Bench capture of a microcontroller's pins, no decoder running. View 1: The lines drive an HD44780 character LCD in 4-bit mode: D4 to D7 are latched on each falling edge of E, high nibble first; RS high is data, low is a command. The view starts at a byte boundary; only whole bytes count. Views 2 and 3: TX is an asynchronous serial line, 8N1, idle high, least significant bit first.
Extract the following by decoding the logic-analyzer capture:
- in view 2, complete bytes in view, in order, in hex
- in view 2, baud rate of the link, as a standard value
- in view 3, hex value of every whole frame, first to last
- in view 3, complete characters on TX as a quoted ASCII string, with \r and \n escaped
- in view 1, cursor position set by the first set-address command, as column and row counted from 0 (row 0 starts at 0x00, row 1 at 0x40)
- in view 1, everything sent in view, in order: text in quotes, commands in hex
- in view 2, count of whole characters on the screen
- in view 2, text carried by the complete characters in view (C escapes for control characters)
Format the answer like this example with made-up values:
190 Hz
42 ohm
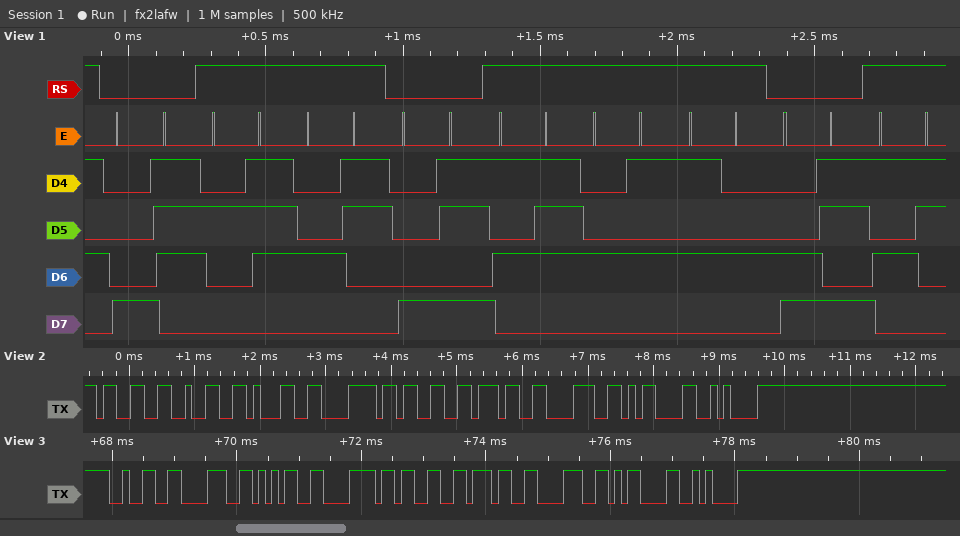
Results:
33 32 31 78 33 37 38 0D 0A
9600 baud
32 38 35 78 33 37 38 0D 0A
"285x378\r\n"
column 7, row 0
0x87 "'C" 0x8B "WET" 0xCB "S"
9
"321x378\r\n"
